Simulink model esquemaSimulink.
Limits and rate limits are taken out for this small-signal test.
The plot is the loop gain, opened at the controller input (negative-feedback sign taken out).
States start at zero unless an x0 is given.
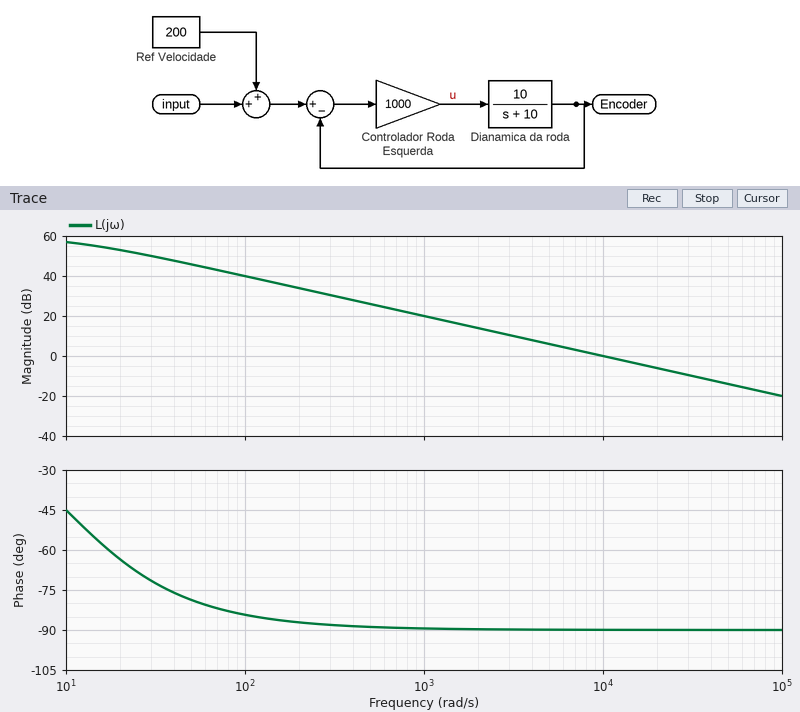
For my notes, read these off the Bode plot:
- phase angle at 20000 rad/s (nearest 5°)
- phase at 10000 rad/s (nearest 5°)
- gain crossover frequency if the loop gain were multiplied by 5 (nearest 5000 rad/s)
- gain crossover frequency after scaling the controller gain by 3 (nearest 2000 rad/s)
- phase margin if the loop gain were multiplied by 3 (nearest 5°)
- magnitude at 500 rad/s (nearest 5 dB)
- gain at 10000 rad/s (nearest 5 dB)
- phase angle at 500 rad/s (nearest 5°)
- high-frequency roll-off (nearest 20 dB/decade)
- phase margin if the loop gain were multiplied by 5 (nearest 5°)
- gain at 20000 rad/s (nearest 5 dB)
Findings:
-90°
-90°
50000 rad/s
30000 rad/s
90°
25 dB
0 dB
-90°
-20 dB/decade
90°
-5 dB
